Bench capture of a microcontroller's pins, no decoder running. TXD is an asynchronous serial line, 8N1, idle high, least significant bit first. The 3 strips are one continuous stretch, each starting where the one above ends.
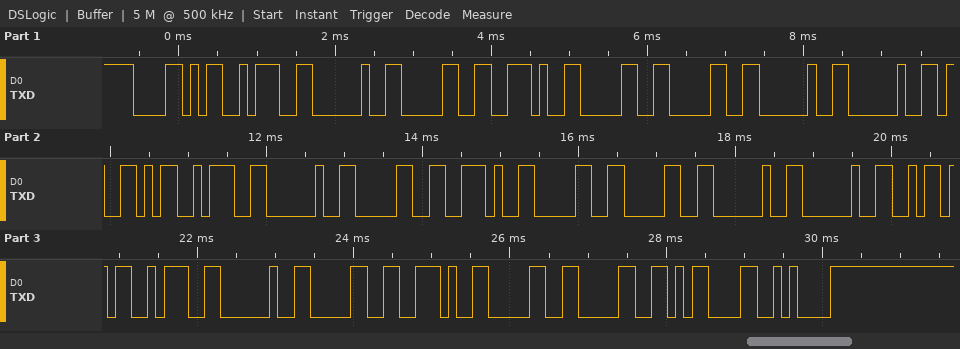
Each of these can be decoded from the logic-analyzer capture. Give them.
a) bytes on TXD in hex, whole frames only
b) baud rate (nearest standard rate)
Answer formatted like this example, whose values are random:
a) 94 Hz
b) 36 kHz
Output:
a) 58 3A 20 30 2E 30 30 20 20 59 3A 20 30 2E 30 30 20 20 5A 3A 20 30 2E 30 30 0D 0A
b) 9600 baud
